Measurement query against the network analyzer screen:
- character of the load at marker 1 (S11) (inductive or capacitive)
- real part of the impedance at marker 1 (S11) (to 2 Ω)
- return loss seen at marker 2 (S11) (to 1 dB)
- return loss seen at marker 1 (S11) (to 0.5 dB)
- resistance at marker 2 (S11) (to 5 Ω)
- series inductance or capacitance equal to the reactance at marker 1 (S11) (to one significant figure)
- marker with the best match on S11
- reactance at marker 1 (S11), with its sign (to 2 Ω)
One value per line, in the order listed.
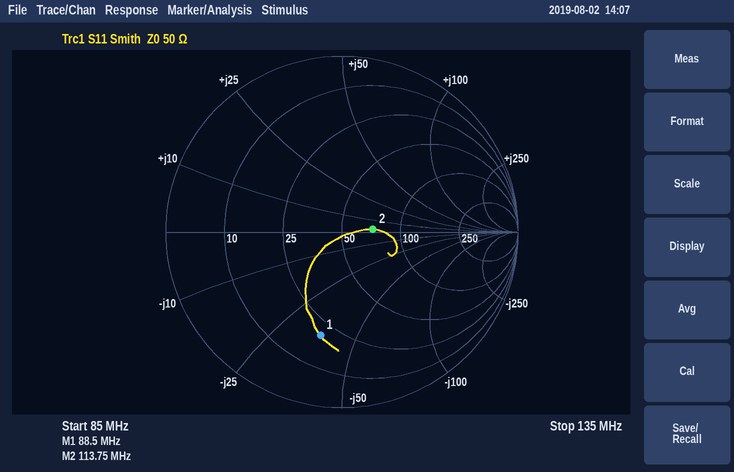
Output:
capacitive
20 Ω
15 dB
4.5 dB
70 Ω
50 pF
marker 2
-36 Ω
